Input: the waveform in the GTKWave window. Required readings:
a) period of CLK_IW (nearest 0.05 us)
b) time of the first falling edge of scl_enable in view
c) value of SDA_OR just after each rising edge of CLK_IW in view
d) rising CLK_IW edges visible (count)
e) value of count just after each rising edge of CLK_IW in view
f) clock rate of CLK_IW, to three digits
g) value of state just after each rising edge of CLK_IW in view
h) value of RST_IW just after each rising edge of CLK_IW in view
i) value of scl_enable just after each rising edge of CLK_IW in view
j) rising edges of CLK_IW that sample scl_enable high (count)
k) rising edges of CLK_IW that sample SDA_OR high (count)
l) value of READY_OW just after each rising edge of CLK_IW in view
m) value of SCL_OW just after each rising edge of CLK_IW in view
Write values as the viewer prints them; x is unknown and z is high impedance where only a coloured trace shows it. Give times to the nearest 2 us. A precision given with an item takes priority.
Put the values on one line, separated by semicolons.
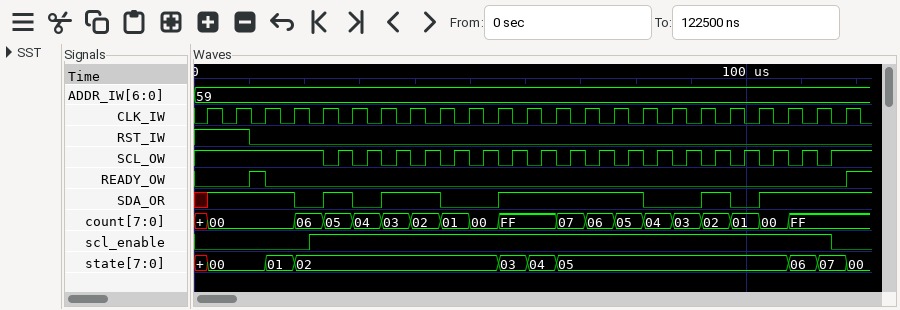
5.25 us; 116 us; 1 1 1 0 1 0 1 1 0 0 1 1 1 1 1 0 0 1 0 1 1 1 1; 23; 00, 00, 00, 06, 05, 04, 03, 02, 01, 00, FF, FF, 07, 06, 05, 04, 03, 02, 01, 00, FF, FF, FF; 190 kHz; 00, 00, 01, 02, 02, 02, 02, 02, 02, 02, 03, 04, 05, 05, 05, 05, 05, 05, 05, 05, 06, 07, 00; 1 1 0 0 0 0 0 0 0 0 0 0 0 0 0 0 0 0 0 0 0 0 0; 0 0 0 0 1 1 1 1 1 1 1 1 1 1 1 1 1 1 1 1 1 1 0; 18; 15; 0 0 0 0 0 0 0 0 0 0 0 0 0 0 0 0 0 0 0 0 0 0 1; 1 1 1 1 0 0 0 0 0 0 0 0 0 0 0 0 0 0 0 0 0 0 1
